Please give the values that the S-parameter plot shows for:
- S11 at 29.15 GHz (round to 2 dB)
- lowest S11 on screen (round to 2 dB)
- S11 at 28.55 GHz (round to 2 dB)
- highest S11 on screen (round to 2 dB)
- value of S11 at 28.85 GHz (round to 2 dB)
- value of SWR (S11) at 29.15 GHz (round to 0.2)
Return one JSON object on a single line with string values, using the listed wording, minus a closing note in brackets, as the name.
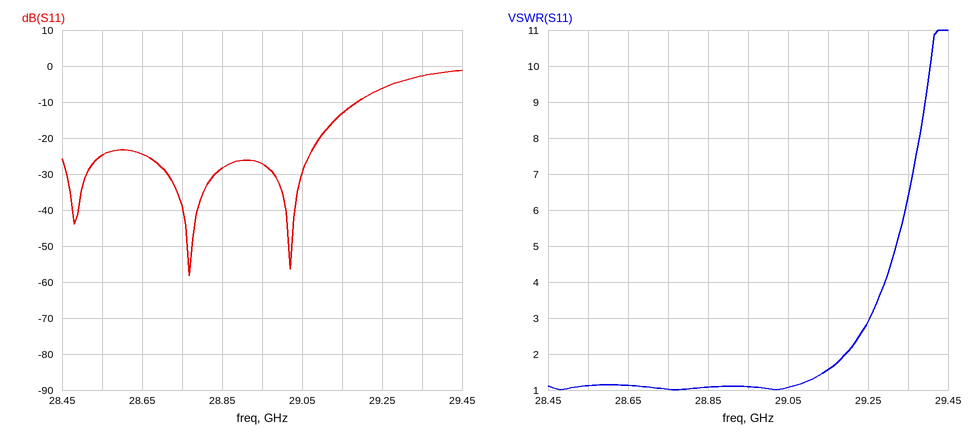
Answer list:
{"S11 at 29.15 GHz": "-14 dB", "lowest S11 on screen": "-58 dB", "S11 at 28.55 GHz": "-24 dB", "highest S11 on screen": "-2 dB", "value of S11 at 28.85 GHz": "-28 dB", "value of SWR (S11) at 29.15 GHz": "1.6"}
